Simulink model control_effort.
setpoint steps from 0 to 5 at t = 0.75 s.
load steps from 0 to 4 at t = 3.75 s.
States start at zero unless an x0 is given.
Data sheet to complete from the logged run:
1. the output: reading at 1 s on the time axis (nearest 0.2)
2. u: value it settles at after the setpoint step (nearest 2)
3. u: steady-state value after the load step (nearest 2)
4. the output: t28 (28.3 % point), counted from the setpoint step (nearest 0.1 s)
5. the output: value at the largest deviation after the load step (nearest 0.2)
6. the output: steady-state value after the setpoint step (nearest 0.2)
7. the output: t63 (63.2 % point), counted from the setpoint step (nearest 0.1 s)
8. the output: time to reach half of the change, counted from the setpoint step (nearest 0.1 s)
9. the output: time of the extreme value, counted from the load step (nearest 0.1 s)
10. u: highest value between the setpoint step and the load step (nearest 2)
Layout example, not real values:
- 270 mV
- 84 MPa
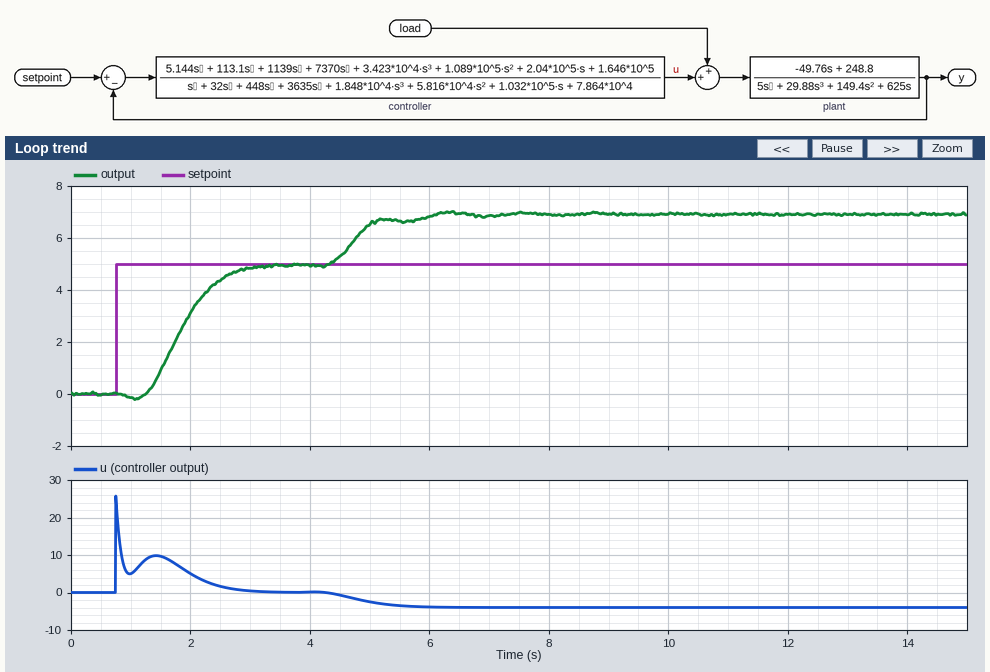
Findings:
- -0.2
- 0
- -4
- 0.9 s
- 7.0
- 5.0
- 1.3 s
- 1.1 s
- 2.6 s
- 26
